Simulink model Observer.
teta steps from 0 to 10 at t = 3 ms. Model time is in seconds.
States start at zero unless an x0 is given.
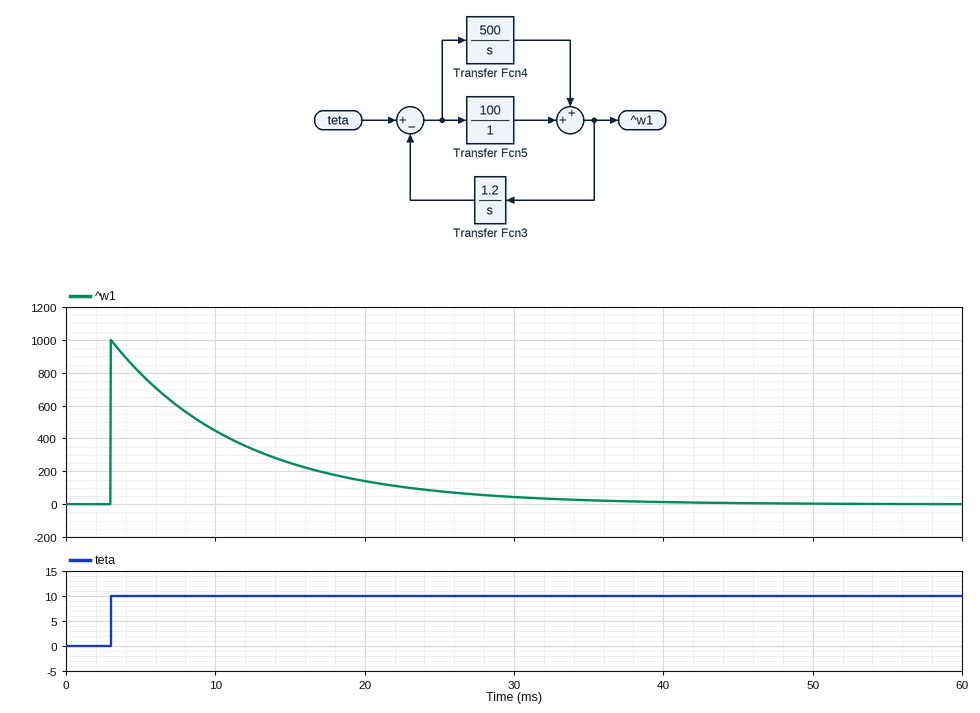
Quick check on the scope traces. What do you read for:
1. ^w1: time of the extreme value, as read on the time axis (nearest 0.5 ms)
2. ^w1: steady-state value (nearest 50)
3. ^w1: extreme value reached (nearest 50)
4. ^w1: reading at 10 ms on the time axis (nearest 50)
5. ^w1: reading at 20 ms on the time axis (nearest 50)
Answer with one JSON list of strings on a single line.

["3.0 ms", "0", "1000", "450", "150"]
